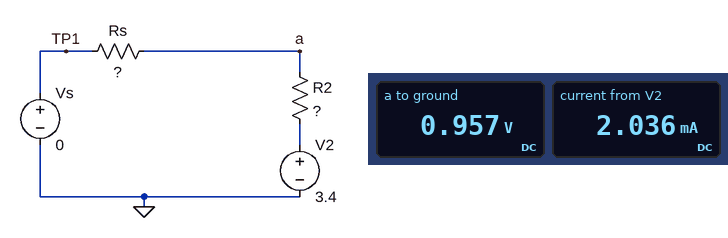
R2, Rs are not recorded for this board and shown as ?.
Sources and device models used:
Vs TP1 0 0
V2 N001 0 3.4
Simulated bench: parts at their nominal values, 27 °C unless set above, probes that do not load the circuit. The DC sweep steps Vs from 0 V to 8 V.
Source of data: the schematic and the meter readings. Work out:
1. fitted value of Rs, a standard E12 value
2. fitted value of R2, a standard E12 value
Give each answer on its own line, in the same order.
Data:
470 Ω
1.2 kΩ
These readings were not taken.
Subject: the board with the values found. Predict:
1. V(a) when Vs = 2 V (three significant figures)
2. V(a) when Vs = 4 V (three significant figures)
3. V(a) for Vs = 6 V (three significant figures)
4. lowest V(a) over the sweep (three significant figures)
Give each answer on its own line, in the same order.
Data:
2.39 V
3.83 V
5.27 V
957 mV
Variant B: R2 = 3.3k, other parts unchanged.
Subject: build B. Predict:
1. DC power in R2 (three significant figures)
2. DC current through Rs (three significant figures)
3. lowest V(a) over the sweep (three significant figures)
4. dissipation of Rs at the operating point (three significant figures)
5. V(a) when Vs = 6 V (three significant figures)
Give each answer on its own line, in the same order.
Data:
2.68 mW
902 µA
424 mV
382 µW
5.68 V
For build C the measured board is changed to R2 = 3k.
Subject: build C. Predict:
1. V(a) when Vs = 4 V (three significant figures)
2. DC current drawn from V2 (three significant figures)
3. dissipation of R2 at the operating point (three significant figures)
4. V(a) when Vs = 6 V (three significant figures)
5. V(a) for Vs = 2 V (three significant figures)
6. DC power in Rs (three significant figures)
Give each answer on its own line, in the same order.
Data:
3.92 V
980 µA
2.88 mW
5.65 V
2.19 V
451 µW
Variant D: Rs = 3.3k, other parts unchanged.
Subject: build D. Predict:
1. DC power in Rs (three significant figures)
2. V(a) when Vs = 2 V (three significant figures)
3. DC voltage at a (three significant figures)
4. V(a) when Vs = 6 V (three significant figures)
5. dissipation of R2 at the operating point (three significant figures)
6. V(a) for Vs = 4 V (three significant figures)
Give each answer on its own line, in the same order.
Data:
1.88 mW
3.03 V
2.49 V
4.09 V
685 µW
3.56 V
